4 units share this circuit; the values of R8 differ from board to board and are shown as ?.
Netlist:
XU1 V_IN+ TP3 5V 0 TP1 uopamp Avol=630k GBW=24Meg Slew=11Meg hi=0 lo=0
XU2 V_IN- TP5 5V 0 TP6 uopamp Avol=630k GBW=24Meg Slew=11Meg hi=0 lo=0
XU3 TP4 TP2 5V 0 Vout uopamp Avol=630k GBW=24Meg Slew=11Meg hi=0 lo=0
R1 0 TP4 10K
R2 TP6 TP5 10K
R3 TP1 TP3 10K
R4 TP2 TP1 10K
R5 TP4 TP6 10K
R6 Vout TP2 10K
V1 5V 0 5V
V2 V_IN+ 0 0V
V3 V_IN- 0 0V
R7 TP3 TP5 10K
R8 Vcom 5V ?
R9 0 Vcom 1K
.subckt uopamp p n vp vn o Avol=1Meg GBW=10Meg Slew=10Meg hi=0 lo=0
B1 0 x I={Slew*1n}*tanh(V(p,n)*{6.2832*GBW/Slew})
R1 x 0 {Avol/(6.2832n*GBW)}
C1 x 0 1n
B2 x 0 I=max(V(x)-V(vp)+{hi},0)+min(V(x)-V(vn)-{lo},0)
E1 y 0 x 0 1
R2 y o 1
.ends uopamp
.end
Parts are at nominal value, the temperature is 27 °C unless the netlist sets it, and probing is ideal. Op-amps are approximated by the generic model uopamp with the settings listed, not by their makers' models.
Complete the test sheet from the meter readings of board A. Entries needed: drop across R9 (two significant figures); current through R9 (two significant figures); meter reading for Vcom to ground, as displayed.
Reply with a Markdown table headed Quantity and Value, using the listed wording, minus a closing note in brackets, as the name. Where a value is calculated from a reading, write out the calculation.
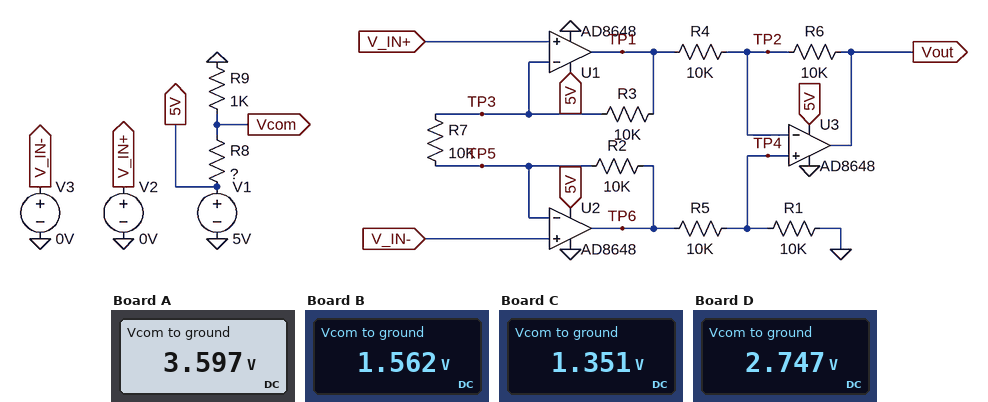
| Quantity | Value |
|---|---|
| drop across R9 | 3.597 V = 3.6 V |
| current through R9 | (3.597 V) / 1 kΩ = 3.6 mA |
| meter reading for Vcom to ground, as displayed | 3.597 V |
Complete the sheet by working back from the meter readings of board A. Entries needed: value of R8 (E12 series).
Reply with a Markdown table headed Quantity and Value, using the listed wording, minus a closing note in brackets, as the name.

| Quantity | Value |
|---|---|
| value of R8 | 390 Ω |
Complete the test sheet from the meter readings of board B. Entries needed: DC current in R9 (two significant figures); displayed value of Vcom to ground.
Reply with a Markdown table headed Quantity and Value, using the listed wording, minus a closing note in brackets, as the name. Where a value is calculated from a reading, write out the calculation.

| Quantity | Value |
|---|---|
| DC current in R9 | (1.562 V) / 1 kΩ = 1.6 mA |
| displayed value of Vcom to ground | 1.562 V |
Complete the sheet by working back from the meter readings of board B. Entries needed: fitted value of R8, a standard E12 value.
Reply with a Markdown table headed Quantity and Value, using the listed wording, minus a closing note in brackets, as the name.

| Quantity | Value |
|---|---|
| fitted value of R8, a standard E12 value | 2.2 kΩ |
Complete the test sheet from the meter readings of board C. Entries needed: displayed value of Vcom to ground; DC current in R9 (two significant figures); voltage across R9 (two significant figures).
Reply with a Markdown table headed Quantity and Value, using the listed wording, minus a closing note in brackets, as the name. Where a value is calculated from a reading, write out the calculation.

| Quantity | Value |
|---|---|
| displayed value of Vcom to ground | 1.351 V |
| DC current in R9 | (1.351 V) / 1 kΩ = 1.4 mA |
| voltage across R9 | 1.351 V = 1.4 V |
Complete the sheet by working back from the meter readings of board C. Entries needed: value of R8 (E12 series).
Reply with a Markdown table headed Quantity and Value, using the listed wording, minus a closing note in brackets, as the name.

| Quantity | Value |
|---|---|
| value of R8 | 2.7 kΩ |
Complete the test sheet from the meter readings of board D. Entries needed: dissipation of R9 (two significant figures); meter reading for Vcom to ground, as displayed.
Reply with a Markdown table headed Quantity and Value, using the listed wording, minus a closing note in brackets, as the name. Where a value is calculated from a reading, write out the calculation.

| Quantity | Value |
|---|---|
| dissipation of R9 | (2.747 V)^2 / 1 kΩ = 7.5 mW |
| meter reading for Vcom to ground, as displayed | 2.747 V |
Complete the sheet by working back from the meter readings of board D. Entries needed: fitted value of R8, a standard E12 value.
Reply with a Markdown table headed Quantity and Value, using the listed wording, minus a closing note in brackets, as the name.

| Quantity | Value |
|---|---|
| fitted value of R8, a standard E12 value | 820 Ω |
